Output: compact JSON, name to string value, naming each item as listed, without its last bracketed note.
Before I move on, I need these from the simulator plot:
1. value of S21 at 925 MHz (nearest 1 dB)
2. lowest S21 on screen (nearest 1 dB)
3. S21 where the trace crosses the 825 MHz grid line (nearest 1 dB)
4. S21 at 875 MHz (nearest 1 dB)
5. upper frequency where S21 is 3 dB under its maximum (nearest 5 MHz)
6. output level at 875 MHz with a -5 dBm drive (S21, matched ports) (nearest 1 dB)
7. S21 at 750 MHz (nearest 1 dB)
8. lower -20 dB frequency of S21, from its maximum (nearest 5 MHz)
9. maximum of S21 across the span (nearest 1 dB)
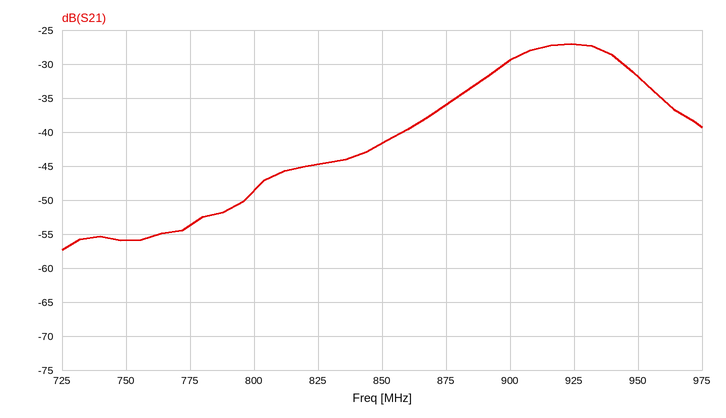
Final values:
{"value of S21 at 925 MHz": "-27 dB", "lowest S21 on screen": "-57 dB", "S21 where the trace crosses the 825 MHz grid line": "-45 dB", "S21 at 875 MHz": "-36 dB", "upper frequency where S21 is 3 dB under its maximum": "945 MHz", "output level at 875 MHz with a -5 dBm drive (S21, matched ports)": "-41 dBm", "S21 at 750 MHz": "-56 dB", "lower -20 dB frequency of S21, from its maximum": "805 MHz", "maximum of S21 across the span": "-27 dB"}
